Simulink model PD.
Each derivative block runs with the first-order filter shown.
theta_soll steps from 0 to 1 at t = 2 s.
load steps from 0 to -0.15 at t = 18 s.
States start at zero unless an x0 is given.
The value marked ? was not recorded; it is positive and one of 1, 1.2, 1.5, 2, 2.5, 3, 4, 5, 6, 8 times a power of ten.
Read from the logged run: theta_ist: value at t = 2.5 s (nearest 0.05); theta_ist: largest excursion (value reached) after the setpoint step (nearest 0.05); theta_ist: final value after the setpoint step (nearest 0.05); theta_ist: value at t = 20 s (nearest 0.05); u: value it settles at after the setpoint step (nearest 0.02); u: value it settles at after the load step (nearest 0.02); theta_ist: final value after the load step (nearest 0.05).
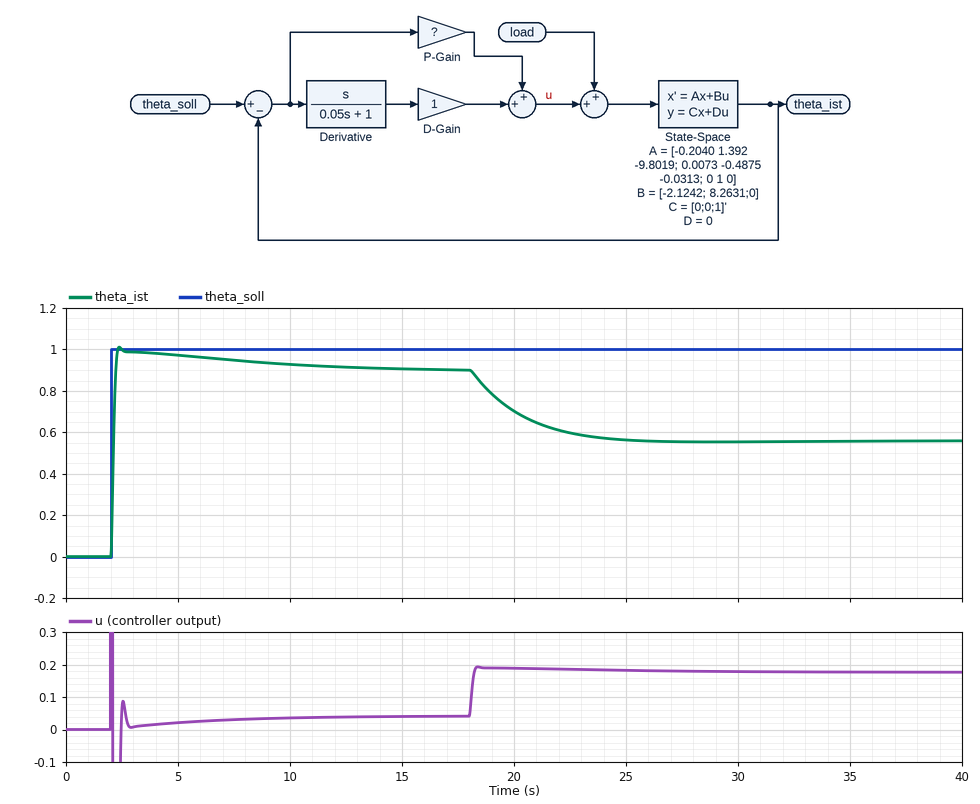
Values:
1.00
1.00
0.90
0.70
0.04
0.18
0.55
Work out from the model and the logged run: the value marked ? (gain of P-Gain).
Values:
0.4
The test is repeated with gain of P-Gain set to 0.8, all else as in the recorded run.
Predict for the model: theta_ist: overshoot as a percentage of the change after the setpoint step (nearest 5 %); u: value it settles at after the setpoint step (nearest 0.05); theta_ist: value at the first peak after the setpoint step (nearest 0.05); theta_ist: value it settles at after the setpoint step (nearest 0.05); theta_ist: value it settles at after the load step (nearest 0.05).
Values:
10 %
0.05
1.05
0.95
0.75
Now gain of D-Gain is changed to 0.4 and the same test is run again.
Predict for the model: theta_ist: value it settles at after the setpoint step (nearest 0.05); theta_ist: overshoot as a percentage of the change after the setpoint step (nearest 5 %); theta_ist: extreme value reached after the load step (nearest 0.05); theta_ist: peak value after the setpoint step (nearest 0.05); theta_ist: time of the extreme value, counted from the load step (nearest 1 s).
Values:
0.90
20 %
0.55
1.05
4 s
